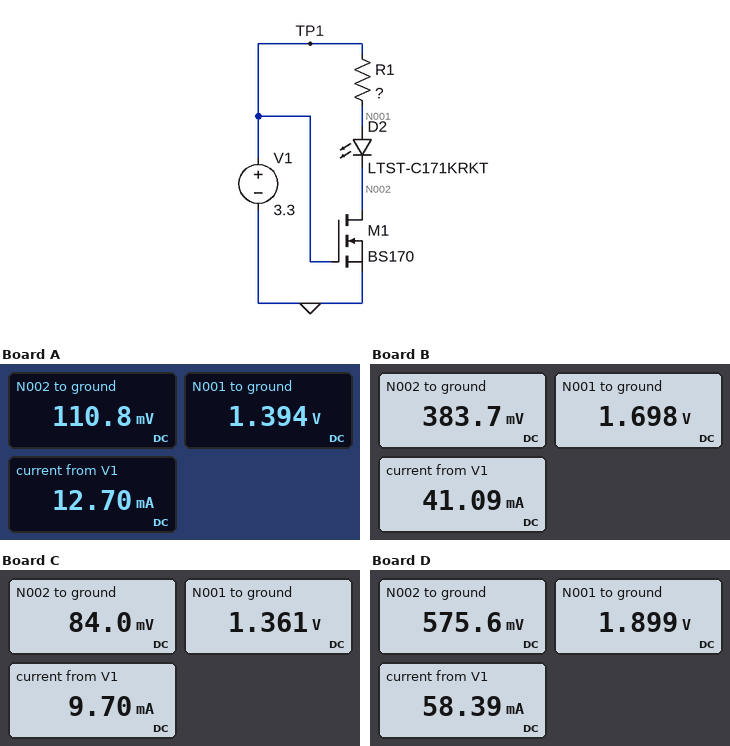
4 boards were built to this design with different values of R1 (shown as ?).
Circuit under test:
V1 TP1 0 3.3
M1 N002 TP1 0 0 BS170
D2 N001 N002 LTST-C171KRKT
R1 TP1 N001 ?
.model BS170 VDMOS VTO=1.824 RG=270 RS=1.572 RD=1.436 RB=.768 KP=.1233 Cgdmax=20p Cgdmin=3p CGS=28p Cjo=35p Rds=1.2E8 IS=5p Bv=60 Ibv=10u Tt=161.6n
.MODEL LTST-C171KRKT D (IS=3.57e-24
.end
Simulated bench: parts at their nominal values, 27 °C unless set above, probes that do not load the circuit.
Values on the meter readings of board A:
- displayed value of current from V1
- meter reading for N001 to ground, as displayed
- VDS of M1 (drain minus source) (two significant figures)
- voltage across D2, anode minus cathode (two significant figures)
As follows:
12.70 mA
1.394 V
110 mV
1.3 V
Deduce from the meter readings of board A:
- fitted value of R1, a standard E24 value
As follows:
150 Ω
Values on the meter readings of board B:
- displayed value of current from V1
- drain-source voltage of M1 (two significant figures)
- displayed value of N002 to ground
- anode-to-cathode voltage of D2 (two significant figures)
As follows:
41.09 mA
380 mV
383.7 mV
1.3 V
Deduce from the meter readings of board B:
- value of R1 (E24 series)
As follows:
39 Ω
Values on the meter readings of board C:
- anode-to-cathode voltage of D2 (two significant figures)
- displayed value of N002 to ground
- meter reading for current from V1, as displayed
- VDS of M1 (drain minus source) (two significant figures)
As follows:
1.3 V
84.0 mV
9.70 mA
84 mV
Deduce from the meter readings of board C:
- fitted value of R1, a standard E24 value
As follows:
200 Ω
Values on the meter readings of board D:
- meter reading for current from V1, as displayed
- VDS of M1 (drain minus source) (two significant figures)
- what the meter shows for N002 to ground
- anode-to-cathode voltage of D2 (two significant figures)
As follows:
58.39 mA
580 mV
575.6 mV
1.3 V
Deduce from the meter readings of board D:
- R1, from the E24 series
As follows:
24 Ω
